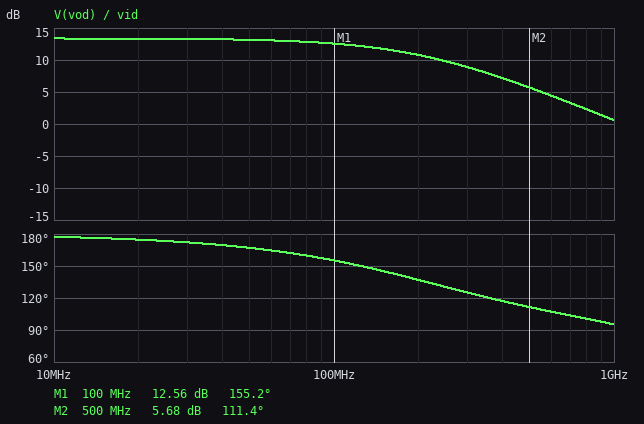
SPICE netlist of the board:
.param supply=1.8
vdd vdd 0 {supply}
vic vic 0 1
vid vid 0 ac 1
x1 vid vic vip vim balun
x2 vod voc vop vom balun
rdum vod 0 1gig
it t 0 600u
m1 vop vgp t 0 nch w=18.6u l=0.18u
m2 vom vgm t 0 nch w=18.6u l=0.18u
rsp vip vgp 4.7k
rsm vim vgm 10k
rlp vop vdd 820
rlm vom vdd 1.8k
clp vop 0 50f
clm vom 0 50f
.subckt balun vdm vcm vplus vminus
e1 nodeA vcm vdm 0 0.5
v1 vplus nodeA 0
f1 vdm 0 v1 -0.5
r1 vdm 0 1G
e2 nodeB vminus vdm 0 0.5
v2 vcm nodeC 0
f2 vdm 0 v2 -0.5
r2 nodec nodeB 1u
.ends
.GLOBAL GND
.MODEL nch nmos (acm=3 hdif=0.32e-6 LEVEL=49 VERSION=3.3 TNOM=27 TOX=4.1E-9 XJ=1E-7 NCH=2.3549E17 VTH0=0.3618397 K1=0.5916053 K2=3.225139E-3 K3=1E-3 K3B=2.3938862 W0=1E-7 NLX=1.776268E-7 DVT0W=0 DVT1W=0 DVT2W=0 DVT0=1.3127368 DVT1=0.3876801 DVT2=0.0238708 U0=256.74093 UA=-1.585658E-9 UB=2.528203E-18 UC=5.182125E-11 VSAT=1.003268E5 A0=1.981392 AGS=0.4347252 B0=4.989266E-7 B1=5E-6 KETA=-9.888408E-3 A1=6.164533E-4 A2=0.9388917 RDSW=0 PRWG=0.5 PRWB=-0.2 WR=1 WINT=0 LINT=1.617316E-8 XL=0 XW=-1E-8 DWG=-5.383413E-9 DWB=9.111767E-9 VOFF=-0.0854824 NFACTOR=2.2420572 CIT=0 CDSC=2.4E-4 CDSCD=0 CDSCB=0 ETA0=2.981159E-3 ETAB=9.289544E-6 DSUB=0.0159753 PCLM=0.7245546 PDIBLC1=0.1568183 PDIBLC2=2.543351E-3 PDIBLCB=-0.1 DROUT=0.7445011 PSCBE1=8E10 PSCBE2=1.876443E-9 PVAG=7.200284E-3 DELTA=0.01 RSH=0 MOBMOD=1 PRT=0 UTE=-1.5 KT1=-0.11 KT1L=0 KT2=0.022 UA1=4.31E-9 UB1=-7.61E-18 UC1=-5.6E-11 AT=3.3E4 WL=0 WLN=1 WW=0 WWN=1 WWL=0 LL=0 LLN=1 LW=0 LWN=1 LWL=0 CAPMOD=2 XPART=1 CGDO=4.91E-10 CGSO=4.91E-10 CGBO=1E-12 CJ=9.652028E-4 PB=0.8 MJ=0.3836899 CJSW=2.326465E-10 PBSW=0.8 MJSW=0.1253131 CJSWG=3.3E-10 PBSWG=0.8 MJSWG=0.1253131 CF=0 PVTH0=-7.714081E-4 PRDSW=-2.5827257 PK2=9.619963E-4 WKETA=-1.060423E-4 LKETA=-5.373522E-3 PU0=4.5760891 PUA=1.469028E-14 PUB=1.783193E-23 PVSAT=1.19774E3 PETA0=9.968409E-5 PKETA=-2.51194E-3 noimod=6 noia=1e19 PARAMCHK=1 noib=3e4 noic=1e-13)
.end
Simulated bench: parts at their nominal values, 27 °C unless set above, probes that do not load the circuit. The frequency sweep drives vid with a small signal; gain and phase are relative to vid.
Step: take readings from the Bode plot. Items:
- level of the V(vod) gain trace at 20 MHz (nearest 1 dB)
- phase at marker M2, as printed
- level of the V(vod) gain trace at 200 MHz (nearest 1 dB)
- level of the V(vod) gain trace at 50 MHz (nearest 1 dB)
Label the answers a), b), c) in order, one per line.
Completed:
a) 13 dB
b) 111.4 deg
c) 11 dB
d) 13 dB
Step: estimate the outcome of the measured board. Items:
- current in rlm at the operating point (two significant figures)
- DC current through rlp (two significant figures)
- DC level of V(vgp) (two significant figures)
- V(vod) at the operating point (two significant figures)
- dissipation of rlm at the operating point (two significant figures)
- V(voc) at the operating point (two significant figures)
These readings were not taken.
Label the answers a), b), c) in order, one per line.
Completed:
a) 290 µA
b) 310 µA
c) 1.0 V
d) 260 mV
e) 150 µW
f) 1.4 V
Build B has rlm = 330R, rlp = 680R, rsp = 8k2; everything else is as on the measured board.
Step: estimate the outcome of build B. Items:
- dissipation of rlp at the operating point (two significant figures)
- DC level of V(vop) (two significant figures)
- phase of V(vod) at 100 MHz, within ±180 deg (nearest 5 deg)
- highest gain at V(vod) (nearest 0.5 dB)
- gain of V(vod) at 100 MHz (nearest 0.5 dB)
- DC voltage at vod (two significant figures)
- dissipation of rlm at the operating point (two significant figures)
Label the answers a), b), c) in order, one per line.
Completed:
a) 59 µW
b) 1.6 V
c) 160 deg
d) 6.0 dB
e) 5.5 dB
f) -100 mV
g) 31 µW
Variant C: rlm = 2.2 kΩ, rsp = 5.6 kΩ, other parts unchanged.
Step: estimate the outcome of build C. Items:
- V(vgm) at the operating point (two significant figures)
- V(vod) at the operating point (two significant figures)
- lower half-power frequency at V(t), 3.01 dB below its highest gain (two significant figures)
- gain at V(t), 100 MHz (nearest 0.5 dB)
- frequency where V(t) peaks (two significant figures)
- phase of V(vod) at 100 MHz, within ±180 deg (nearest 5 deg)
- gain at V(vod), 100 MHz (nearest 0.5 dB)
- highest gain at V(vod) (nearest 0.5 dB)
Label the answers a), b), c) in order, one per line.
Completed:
a) 1.0 V
b) 360 mV
c) 140 MHz
d) -20.5 dB
e) 470 MHz
f) 150 deg
g) 13.5 dB
h) 14.5 dB
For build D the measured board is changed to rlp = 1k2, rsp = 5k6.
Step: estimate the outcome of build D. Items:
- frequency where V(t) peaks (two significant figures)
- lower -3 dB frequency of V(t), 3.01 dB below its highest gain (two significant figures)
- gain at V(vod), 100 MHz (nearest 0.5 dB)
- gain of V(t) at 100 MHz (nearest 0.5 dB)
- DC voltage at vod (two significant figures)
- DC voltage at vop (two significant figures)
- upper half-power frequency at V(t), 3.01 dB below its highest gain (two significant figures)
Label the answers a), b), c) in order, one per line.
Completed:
a) 490 MHz
b) 160 MHz
c) 13.5 dB
d) -24.0 dB
e) 160 mV
f) 1.4 V
g) 1.4 GHz
